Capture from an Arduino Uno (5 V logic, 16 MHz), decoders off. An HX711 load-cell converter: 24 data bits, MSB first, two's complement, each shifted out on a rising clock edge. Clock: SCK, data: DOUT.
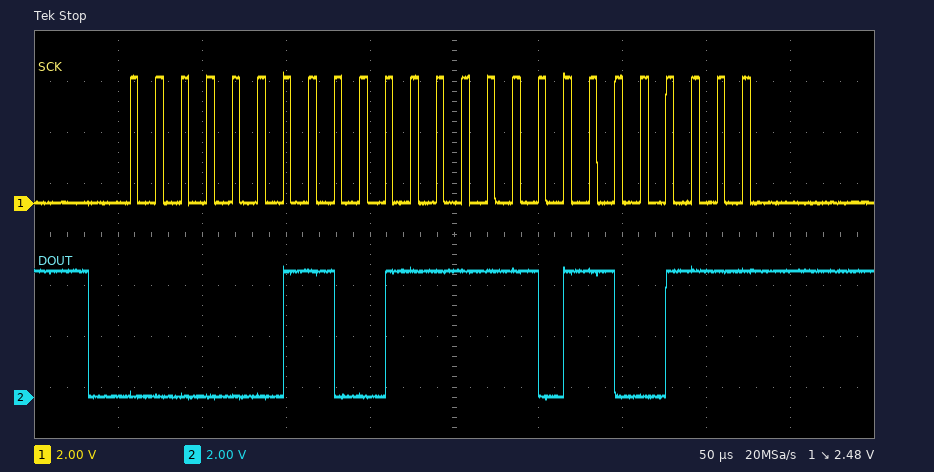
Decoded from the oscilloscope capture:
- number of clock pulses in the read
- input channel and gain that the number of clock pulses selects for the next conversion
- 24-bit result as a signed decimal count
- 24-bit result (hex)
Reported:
25
channel A, gain 128
212839
0x033F67
